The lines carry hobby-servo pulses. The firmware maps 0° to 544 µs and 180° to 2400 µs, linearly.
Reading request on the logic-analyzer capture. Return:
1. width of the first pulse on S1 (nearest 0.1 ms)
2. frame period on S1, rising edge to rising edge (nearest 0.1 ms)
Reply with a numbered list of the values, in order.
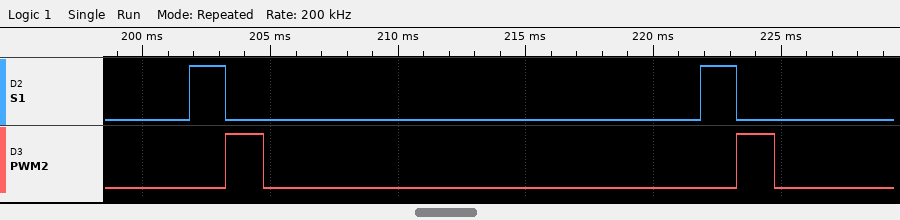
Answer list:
1. 1.4 ms
2. 20.0 ms
